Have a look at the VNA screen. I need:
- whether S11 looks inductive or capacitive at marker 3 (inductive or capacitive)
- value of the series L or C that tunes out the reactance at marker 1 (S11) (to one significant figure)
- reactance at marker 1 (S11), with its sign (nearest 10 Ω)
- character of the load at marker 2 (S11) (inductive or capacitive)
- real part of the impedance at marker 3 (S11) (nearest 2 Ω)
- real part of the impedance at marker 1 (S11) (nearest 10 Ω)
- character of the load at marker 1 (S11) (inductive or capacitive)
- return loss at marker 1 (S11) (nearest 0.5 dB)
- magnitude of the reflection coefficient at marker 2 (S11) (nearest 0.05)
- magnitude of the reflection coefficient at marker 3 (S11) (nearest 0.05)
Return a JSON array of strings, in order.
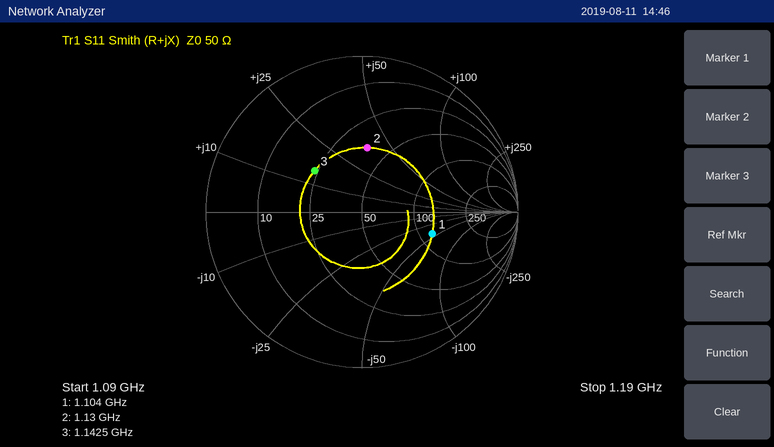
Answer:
["inductive", "6 nH", "-40 Ω", "inductive", "24 Ω", "120 Ω", "capacitive", "6.5 dB", "0.40", "0.40"]
